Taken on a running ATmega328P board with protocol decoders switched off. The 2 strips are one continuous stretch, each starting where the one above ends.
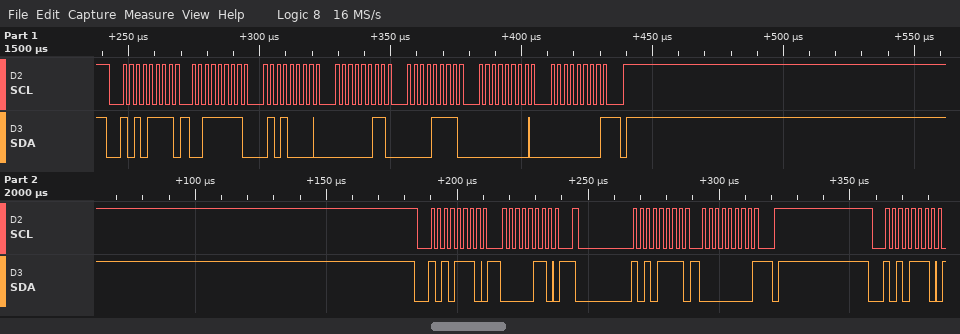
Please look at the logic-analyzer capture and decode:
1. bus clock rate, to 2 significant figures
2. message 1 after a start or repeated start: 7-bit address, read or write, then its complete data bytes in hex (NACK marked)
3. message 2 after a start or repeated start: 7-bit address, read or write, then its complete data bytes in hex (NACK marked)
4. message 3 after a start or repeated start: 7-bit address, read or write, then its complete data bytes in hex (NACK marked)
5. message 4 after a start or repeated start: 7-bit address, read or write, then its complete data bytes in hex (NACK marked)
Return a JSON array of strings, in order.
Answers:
["400 kHz", "0x57 read: 3F 50 03 0F 00 00 NACK", "0x57 write: 06", "0x57 read: 00 NACK", "0x57 write"]
